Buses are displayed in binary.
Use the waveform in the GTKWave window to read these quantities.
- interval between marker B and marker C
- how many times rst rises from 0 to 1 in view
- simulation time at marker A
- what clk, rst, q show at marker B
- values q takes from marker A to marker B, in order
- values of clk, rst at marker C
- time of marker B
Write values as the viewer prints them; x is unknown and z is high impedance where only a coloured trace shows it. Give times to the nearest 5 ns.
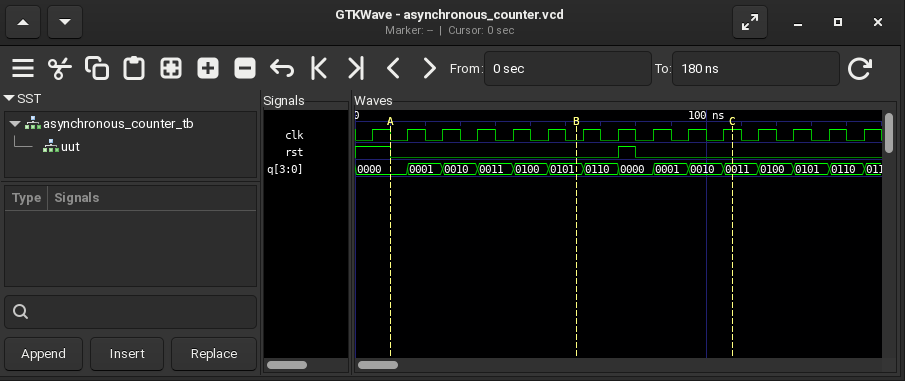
45 ns
1
10 ns
clk=0, rst=0, q=0101
0000, 0001, 0010, 0011, 0100, 0101
clk=1, rst=0
65 ns
